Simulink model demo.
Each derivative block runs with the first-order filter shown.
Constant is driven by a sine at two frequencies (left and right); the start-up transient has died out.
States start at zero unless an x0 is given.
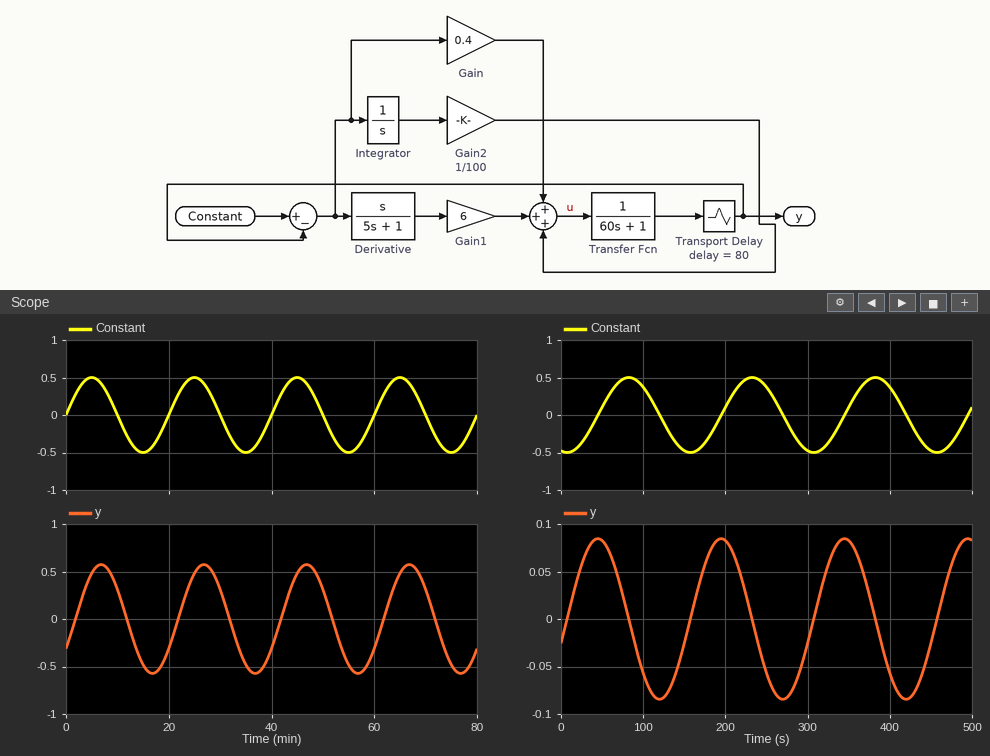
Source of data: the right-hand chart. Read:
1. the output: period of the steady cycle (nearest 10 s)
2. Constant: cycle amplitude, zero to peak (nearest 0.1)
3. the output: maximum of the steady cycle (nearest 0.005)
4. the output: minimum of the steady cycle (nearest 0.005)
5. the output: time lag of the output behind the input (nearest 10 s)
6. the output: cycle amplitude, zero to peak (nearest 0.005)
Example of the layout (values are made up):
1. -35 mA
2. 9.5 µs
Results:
1. 150 s
2. 0.5
3. 0.085
4. -0.085
5. 110 s
6. 0.085
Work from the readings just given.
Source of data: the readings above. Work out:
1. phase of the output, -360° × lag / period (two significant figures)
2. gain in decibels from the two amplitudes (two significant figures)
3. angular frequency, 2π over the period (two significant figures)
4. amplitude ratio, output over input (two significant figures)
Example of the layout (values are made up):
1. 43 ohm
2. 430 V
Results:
1. -260°
2. -15 dB
3. 0.042 rad/s
4. 0.17
